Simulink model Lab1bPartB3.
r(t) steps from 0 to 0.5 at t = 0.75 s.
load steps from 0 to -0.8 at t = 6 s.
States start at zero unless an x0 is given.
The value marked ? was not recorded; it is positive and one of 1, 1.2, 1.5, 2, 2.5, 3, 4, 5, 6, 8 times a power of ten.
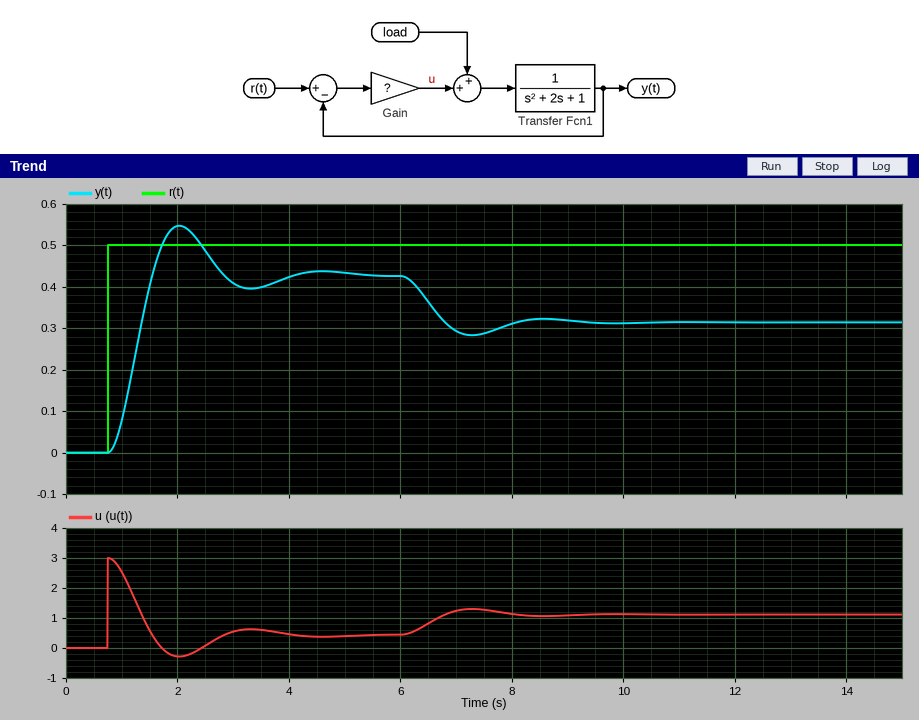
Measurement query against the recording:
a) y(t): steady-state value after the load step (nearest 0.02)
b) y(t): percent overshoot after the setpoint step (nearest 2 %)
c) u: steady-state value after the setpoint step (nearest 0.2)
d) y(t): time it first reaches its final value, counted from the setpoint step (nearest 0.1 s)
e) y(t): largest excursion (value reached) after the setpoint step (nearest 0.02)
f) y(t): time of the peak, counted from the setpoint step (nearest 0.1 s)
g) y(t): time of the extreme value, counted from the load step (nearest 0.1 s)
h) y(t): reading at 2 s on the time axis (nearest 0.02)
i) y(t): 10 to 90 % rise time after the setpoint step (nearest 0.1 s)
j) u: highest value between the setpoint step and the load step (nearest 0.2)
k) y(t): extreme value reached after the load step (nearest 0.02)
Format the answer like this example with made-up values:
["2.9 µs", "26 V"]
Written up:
["0.32", "28 %", "0.4", "0.8 s", "0.54", "1.3 s", "1.3 s", "0.54", "0.5 s", "3.0", "0.28"]
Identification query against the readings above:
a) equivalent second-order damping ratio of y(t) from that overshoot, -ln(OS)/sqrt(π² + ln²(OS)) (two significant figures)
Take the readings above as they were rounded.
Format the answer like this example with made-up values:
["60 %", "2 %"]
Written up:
["0.38"]
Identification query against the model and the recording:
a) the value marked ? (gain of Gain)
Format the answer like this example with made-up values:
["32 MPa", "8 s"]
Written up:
["6"]
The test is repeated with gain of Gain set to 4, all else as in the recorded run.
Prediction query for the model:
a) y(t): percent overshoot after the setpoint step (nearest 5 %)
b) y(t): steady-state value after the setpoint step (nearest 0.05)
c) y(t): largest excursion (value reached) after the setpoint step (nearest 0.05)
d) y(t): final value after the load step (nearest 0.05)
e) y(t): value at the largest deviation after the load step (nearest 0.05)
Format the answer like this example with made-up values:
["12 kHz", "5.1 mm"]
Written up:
["20 %", "0.40", "0.50", "0.25", "0.20"]
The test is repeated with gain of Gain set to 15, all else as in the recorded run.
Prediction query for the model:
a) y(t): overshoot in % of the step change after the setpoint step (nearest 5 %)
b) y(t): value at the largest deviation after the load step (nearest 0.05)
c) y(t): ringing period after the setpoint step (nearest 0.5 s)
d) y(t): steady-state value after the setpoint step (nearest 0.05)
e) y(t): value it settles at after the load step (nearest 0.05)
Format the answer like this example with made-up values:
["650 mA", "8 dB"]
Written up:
["45 %", "0.40", "1.5 s", "0.45", "0.40"]
